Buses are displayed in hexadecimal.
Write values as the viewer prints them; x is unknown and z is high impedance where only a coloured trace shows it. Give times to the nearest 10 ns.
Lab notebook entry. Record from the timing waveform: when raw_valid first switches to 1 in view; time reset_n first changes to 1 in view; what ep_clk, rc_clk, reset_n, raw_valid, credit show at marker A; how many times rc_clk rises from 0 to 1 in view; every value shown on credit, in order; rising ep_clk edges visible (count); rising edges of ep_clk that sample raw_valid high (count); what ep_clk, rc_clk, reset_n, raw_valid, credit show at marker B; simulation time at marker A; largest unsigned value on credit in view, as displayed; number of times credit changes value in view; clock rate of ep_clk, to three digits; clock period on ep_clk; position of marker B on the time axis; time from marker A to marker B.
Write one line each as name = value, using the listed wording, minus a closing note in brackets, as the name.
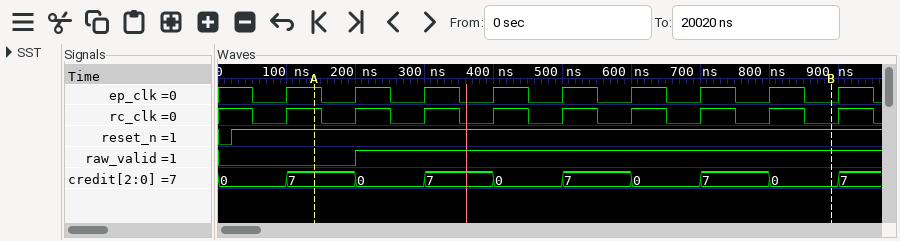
when raw_valid first switches to 1 in view = 200 ns
time reset_n first changes to 1 in view = 20 ns
what ep_clk, rc_clk, reset_n, raw_valid, credit show at marker A = ep_clk=1, rc_clk=1, reset_n=1, raw_valid=0, credit=7
how many times rc_clk rises from 0 to 1 in view = 9
every value shown on credit, in order = 0, 7, 0, 7, 0, 7, 0, 7, 0, 7
rising ep_clk edges visible = 9
rising edges of ep_clk that sample raw_valid high = 7
what ep_clk, rc_clk, reset_n, raw_valid, credit show at marker B = ep_clk=0, rc_clk=0, reset_n=1, raw_valid=1, credit=0
simulation time at marker A = 140 ns
largest unsigned value on credit in view, as displayed = 7
number of times credit changes value in view = 9
clock rate of ep_clk, to three digits = 10.0 MHz
clock period on ep_clk = 100 ns
position of marker B on the time axis = 890 ns
time from marker A to marker B = 750 ns
